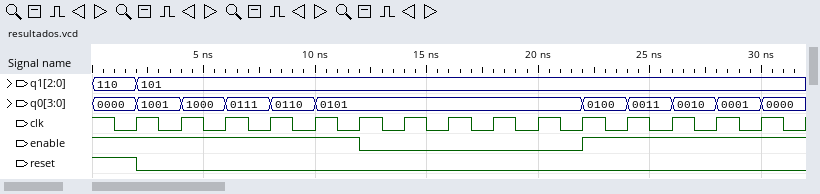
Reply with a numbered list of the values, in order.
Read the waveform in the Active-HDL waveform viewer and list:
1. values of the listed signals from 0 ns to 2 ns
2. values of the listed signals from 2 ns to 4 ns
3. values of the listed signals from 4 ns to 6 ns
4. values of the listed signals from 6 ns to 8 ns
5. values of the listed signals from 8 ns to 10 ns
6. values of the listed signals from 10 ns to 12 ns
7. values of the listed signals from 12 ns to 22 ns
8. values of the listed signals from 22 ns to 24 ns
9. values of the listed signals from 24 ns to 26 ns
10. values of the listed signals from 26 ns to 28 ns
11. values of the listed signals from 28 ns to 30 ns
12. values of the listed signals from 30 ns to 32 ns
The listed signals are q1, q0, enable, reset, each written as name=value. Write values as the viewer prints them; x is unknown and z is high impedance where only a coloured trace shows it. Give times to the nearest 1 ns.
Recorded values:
1. q1=110, q0=0000, enable=1, reset=1
2. q1=101, q0=1001, enable=1, reset=0
3. q1=101, q0=1000, enable=1, reset=0
4. q1=101, q0=0111, enable=1, reset=0
5. q1=101, q0=0110, enable=1, reset=0
6. q1=101, q0=0101, enable=1, reset=0
7. q1=101, q0=0101, enable=0, reset=0
8. q1=101, q0=0100, enable=1, reset=0
9. q1=101, q0=0011, enable=1, reset=0
10. q1=101, q0=0010, enable=1, reset=0
11. q1=101, q0=0001, enable=1, reset=0
12. q1=101, q0=0000, enable=1, reset=0
